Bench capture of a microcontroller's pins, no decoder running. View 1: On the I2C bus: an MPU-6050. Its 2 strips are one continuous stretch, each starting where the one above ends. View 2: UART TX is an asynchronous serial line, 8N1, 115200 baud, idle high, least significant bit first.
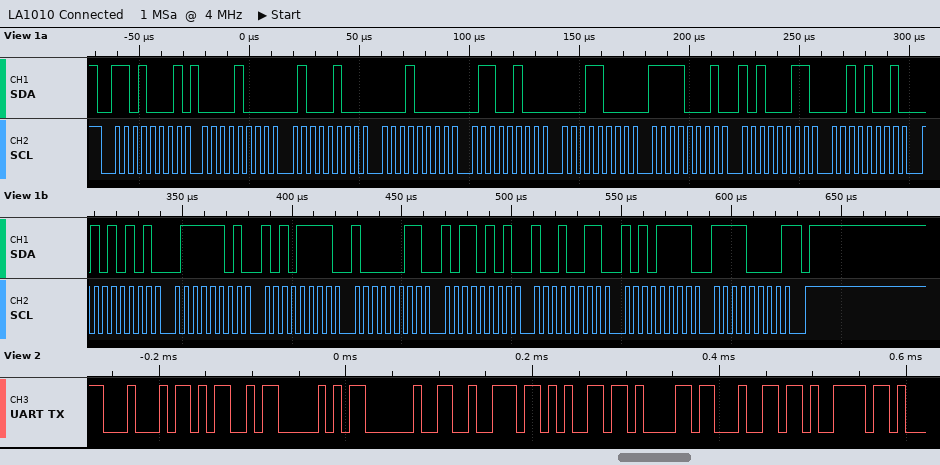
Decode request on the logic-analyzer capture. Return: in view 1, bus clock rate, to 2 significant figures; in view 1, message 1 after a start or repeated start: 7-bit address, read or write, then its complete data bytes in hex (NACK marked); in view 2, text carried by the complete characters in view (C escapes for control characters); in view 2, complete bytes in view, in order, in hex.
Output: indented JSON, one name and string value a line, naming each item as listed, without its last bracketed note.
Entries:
{
  "in view 1, bus clock rate, to 2 significant figures": "250 kHz",
  "in view 1, message 1 after a start or repeated start: 7-bit address, read or write, then its complete data bytes in hex": "0x68 read: 08 44 10 64 18 F1 A3 29 55 7D AF 83 B5 93 AF F0 NACK",
  "in view 2, text carried by the complete characters in view": "\"DMP ready\"",
  "in view 2, complete bytes in view, in order, in hex": "44 4D 50 20 72 65 61 64 79"
}
